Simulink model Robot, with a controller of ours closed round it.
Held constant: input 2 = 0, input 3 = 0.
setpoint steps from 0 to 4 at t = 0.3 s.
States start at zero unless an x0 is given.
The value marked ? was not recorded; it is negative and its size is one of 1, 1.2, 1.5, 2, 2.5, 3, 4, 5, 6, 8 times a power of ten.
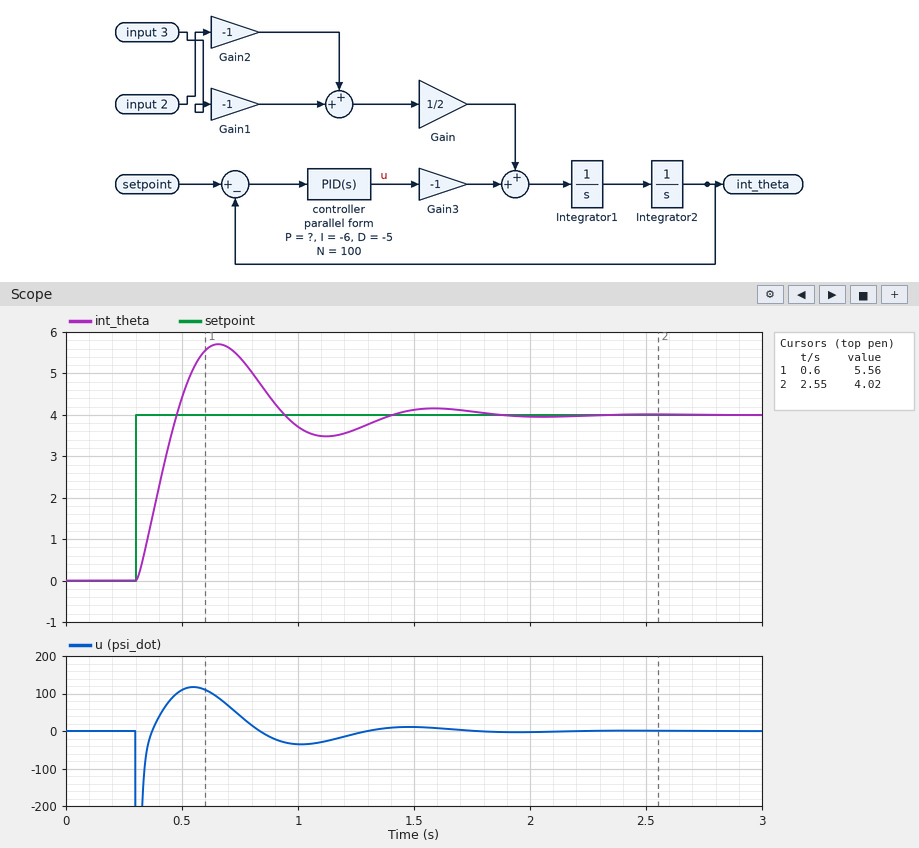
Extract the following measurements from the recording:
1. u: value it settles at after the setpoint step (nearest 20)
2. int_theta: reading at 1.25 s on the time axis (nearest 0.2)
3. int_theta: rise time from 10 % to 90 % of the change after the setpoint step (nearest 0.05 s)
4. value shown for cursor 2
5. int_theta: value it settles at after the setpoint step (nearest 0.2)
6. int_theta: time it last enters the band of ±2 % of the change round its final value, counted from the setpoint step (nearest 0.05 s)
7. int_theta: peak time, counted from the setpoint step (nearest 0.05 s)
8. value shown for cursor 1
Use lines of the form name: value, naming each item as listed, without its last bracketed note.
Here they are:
u: value it settles at after the setpoint step: 0
int_theta: reading at 1.25 s on the time axis: 3.6
int_theta: rise time from 10 % to 90 % of the change after the setpoint step: 0.15 s
value shown for cursor 2: 4.02
int_theta: value it settles at after the setpoint step: 4.0
int_theta: time it last enters the band of ±2 % of the change round its final value, counted from the setpoint step: 1.45 s
int_theta: peak time, counted from the setpoint step: 0.35 s
value shown for cursor 1: 5.56
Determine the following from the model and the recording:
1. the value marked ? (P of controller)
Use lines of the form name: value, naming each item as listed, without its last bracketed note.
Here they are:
the value marked ?: -50
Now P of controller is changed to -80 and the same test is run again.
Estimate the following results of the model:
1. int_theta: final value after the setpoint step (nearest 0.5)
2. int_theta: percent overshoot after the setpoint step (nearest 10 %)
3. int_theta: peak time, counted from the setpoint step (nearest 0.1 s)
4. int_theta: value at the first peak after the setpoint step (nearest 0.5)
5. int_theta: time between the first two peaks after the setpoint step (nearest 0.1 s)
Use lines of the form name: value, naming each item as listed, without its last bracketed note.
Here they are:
int_theta: final value after the setpoint step: 4.0
int_theta: percent overshoot after the setpoint step: 50 %
int_theta: peak time, counted from the setpoint step: 0.3 s
int_theta: value at the first peak after the setpoint step: 6.0
int_theta: time between the first two peaks after the setpoint step: 0.7 s
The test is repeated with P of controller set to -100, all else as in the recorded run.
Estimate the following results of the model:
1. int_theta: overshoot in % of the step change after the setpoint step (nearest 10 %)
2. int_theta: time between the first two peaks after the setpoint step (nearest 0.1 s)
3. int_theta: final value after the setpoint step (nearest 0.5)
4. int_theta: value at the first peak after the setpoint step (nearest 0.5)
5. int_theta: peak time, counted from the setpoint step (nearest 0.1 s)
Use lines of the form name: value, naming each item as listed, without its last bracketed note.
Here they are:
int_theta: overshoot in % of the step change after the setpoint step: 50 %
int_theta: time between the first two peaks after the setpoint step: 0.6 s
int_theta: final value after the setpoint step: 4.0
int_theta: value at the first peak after the setpoint step: 6.0
int_theta: peak time, counted from the setpoint step: 0.3 s
